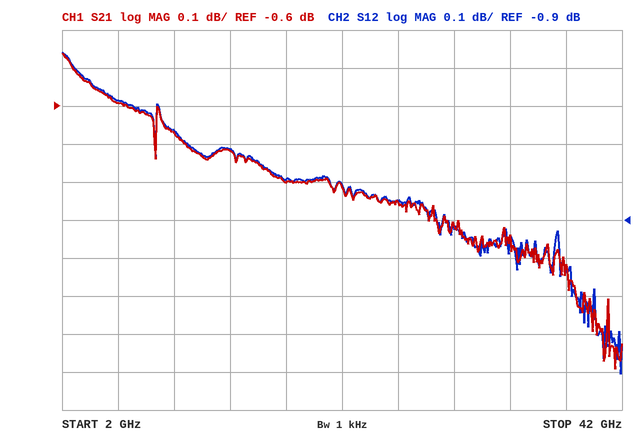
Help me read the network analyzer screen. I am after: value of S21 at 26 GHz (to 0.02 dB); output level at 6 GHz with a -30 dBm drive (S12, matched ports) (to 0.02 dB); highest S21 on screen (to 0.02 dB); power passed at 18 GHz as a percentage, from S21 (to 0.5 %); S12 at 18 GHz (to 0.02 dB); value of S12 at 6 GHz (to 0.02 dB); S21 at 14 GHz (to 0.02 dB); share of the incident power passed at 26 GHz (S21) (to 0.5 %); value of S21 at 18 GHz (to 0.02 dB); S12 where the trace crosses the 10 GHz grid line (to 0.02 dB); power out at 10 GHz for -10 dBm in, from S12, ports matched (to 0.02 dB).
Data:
-0.86 dB
-30.58 dBm
-0.46 dB
83.0 %
-0.80 dB
-0.58 dB
-0.72 dB
82.0 %
-0.80 dB
-0.66 dB
-10.66 dBm
